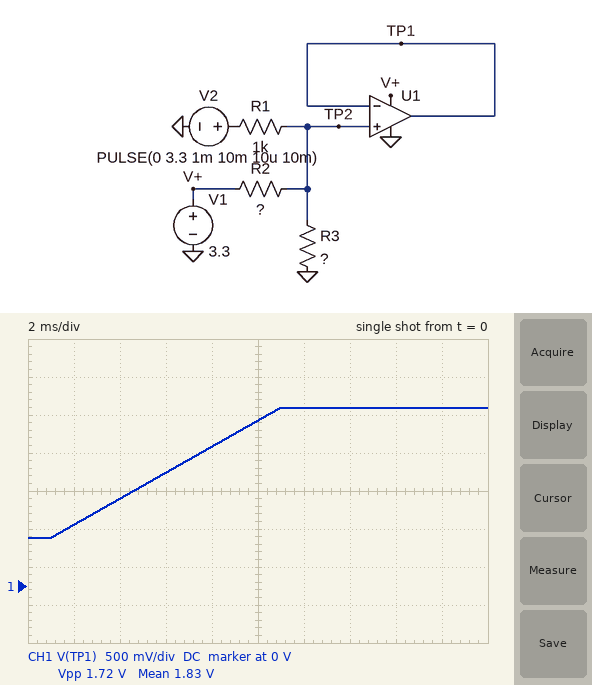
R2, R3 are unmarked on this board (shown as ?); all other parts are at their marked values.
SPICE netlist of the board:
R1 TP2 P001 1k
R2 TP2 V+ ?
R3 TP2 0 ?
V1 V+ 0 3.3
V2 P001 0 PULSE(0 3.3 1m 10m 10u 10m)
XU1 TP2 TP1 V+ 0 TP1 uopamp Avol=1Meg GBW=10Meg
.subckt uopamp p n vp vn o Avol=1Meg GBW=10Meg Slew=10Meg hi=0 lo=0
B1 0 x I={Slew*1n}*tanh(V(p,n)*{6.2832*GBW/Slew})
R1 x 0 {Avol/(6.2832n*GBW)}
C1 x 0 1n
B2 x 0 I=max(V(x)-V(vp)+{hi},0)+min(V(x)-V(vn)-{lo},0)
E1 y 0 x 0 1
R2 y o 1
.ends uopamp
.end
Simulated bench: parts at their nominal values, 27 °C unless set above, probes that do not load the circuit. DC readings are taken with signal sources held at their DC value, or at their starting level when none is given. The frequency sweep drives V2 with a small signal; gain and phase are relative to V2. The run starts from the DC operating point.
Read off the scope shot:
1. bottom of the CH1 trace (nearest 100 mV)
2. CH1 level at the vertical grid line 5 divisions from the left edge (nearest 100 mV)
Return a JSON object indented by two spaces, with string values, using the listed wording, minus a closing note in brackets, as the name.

{
  "bottom of the CH1 trace": "600 mV",
  "CH1 level at the vertical grid line 5 divisions from the left edge": "2.2 V"
}
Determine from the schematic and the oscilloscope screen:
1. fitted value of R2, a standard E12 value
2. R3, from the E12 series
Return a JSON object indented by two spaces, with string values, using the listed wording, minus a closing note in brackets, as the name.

{
  "fitted value of R2, a standard E12 value": "2.7 kΩ",
  "R3, from the E12 series": "1.8 kΩ"
}
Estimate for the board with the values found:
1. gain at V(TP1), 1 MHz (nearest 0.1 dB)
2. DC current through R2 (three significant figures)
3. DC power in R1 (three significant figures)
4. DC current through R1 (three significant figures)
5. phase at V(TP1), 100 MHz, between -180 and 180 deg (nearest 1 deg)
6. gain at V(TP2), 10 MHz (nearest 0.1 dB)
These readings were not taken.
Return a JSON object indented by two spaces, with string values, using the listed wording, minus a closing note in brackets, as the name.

{
  "gain at V(TP1), 1 MHz": "-5.7 dB",
  "DC current through R2": "987 µA",
  "DC power in R1": "403 µW",
  "DC current through R1": "635 µA",
  "phase at V(TP1), 100 MHz, between -180 and 180 deg": "-84 deg",
  "gain at V(TP2), 10 MHz": "-5.7 dB"
}
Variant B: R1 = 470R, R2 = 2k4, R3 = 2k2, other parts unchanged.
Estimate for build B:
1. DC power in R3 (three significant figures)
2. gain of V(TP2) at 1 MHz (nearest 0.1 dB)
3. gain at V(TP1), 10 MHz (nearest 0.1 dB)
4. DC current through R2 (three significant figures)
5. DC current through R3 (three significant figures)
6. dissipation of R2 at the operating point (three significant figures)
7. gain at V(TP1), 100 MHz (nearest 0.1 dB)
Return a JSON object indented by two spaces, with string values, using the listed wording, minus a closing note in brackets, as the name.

{
  "DC power in R3": "95.6 µW",
  "gain of V(TP2) at 1 MHz": "-3.0 dB",
  "gain at V(TP1), 10 MHz": "-6.0 dB",
  "DC current through R2": "1.18 mA",
  "DC current through R3": "208 µA",
  "dissipation of R2 at the operating point": "3.36 mW",
  "gain at V(TP1), 100 MHz": "-23.0 dB"
}
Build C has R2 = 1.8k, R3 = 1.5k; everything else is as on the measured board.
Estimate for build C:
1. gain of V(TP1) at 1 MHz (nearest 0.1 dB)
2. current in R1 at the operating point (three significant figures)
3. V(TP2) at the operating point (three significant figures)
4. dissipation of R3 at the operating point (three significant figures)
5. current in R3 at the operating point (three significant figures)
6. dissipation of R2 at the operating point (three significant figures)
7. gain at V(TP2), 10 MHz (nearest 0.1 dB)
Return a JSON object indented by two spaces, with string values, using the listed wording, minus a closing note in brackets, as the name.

{
  "gain of V(TP1) at 1 MHz": "-7.0 dB",
  "current in R1 at the operating point": "825 µA",
  "V(TP2) at the operating point": "825 mV",
  "dissipation of R3 at the operating point": "454 µW",
  "current in R3 at the operating point": "550 µA",
  "dissipation of R2 at the operating point": "3.40 mW",
  "gain at V(TP2), 10 MHz": "-6.9 dB"
}
